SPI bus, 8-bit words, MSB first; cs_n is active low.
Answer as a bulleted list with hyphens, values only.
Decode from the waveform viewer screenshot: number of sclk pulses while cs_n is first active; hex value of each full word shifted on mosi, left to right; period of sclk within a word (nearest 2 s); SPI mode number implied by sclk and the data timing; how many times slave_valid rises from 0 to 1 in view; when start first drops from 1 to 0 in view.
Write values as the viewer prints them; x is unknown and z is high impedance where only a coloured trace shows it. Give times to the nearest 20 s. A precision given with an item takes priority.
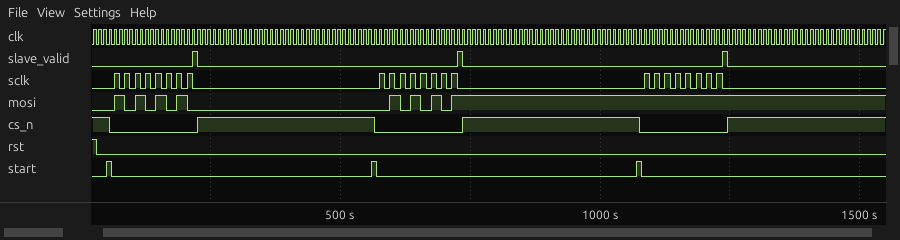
- 8
- AA, 55, FF
- 20 s
- 1
- 3
- 60 s
